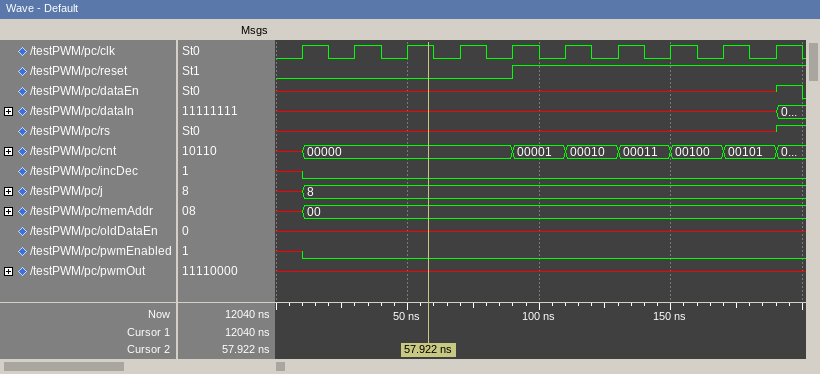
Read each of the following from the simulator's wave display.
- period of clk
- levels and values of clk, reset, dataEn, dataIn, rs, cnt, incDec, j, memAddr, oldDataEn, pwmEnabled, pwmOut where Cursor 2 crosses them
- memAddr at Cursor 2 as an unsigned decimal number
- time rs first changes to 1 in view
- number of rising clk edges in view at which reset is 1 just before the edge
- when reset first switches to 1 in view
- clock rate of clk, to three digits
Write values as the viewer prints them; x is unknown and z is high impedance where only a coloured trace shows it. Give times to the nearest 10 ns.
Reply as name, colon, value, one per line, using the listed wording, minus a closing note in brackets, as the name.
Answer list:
period of clk: 20 ns
levels and values of clk, reset, dataEn, dataIn, rs, cnt, incDec, j, memAddr, oldDataEn, pwmEnabled, pwmOut where Cursor 2 crosses them: clk=1, reset=0, dataEn=x, dataIn=x, rs=x, cnt=00000, incDec=0, j=8, memAddr=00, oldDataEn=x, pwmEnabled=0, pwmOut=x
memAddr at Cursor 2 as an unsigned decimal number: 0
time rs first changes to 1 in view: 190 ns
number of rising clk edges in view at which reset is 1 just before the edge: 5
when reset first switches to 1 in view: 90 ns
clock rate of clk, to three digits: 50.0 MHz
